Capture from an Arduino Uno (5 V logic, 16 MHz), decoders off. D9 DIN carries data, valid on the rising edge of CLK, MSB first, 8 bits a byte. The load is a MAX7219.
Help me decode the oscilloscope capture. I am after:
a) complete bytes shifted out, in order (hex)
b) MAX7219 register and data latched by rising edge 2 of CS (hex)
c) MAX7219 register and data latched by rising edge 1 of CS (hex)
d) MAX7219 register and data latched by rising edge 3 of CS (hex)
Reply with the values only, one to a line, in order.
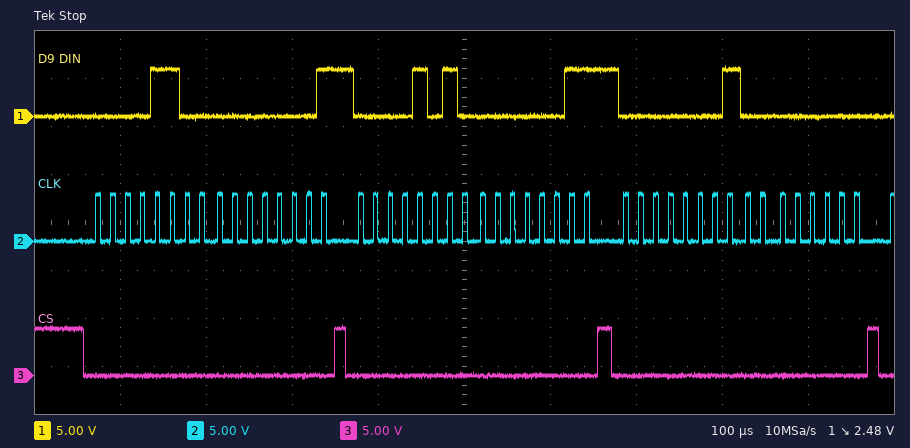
0C 01 0A 03 01 00
register 0xA, data 0x03
register 0xC, data 0x01
register 0x1, data 0x00
